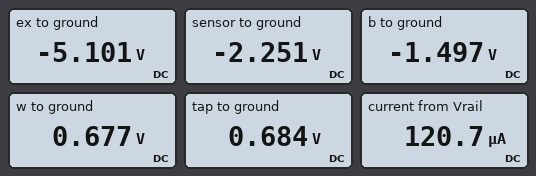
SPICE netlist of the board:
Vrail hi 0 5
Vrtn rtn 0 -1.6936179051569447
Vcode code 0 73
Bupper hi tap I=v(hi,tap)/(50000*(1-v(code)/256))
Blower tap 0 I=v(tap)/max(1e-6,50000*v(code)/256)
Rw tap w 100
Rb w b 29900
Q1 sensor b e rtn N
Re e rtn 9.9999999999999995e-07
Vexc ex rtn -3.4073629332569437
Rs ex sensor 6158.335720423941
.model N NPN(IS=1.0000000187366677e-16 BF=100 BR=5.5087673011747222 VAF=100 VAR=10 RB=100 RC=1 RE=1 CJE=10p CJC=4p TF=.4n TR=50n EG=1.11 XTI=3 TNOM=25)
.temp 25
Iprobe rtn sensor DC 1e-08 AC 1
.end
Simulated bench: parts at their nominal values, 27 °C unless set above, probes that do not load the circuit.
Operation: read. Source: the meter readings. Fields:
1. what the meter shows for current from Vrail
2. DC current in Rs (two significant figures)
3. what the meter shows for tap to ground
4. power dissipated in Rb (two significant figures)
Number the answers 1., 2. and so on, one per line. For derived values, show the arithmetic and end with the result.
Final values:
1. 120.7 µA
2. (-2.251 V - (-5.101 V)) / 6.158 kΩ = 460 µA
3. 0.684 V
4. (677 mV - (-1.497 V))^2 / 29.9 kΩ = 160 µW
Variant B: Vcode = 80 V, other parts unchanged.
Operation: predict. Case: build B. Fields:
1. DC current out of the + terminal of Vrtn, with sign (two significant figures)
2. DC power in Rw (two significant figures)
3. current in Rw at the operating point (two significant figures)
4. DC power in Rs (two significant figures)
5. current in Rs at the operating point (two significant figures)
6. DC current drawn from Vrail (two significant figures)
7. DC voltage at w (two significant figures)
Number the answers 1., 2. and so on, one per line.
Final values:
1. -74 µA
2. 550 nW
3. 74 µA
4. 1.4 mW
5. 470 µA
6. 120 µA
7. 760 mV
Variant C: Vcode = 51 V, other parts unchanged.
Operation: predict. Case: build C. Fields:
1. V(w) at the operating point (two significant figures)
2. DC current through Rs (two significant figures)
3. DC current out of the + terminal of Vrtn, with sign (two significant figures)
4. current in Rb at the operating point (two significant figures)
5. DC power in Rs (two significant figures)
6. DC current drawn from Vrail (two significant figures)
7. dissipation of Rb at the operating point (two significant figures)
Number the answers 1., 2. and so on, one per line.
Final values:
1. 440 mV
2. 440 µA
3. -69 µA
4. 69 µA
5. 1.2 mW
6. 110 µA
7. 140 µW
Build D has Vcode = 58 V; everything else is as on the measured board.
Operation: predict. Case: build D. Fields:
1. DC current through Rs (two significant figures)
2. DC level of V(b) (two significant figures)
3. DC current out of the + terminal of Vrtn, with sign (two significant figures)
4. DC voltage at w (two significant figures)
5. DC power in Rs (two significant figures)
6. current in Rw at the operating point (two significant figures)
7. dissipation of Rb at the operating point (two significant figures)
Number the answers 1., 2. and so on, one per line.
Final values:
1. 450 µA
2. -1.6 V
3. -70 µA
4. 510 mV
5. 1.2 mW
6. 70 µA
7. 150 µW
